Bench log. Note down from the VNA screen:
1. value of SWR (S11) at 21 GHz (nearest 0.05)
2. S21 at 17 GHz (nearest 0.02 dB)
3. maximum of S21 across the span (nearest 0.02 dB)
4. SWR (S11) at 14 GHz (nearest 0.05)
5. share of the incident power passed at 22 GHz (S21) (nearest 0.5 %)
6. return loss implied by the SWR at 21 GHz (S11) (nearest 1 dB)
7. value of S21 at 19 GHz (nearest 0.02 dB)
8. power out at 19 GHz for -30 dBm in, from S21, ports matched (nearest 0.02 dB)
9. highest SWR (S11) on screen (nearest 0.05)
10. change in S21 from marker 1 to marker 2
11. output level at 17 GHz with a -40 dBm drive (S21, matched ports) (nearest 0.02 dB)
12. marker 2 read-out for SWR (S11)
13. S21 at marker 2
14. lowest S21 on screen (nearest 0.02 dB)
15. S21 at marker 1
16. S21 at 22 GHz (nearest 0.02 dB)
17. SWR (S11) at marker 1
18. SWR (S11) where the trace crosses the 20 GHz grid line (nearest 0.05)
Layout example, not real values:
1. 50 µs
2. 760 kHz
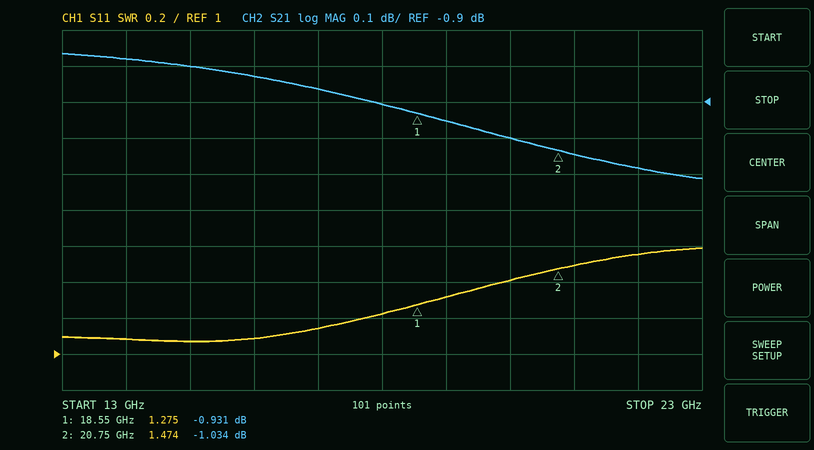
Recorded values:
1. 1.50
2. -0.86 dB
3. -0.76 dB
4. 1.10
5. 78.0 %
6. 14 dB
7. -0.96 dB
8. -30.96 dBm
9. 1.60
10. -0.103 dB
11. -40.86 dBm
12. 1.474
13. -1.034 dB
14. -1.12 dB
15. -0.931 dB
16. -1.08 dB
17. 1.275
18. 1.40
